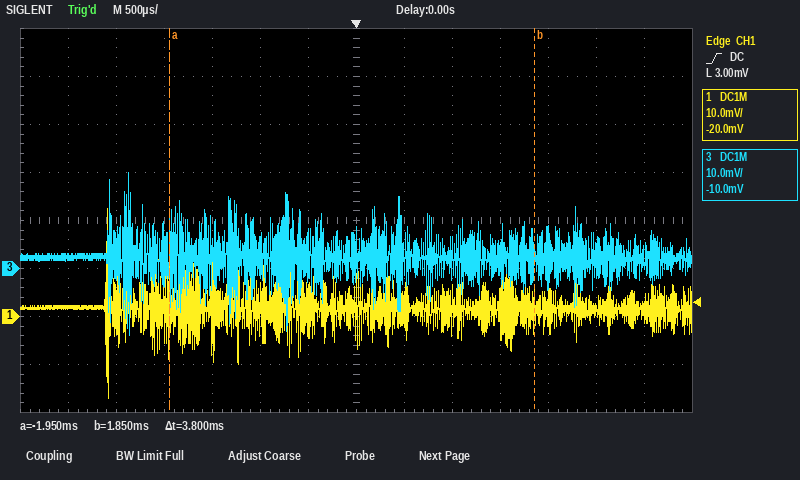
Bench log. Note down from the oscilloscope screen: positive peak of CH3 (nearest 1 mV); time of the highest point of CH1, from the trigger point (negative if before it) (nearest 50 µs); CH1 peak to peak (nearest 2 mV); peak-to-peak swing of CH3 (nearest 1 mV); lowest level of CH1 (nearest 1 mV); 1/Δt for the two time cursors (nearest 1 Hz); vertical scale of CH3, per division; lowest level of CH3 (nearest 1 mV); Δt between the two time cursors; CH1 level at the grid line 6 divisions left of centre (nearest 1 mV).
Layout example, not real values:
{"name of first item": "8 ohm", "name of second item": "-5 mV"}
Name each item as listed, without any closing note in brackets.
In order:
{"positive peak of CH3": "20 mV", "time of the highest point of CH1, from the trigger point (negative if before it)": "-2.60 ms", "CH1 peak to peak": "40 mV", "peak-to-peak swing of CH3": "34 mV", "lowest level of CH1": "-17 mV", "1/Δt for the two time cursors": "263 Hz", "vertical scale of CH3, per division": "10 mV", "lowest level of CH3": "-14 mV", "Δt between the two time cursors": "3.8 ms", "CH1 level at the grid line 6 divisions left of centre": "2 mV"}
